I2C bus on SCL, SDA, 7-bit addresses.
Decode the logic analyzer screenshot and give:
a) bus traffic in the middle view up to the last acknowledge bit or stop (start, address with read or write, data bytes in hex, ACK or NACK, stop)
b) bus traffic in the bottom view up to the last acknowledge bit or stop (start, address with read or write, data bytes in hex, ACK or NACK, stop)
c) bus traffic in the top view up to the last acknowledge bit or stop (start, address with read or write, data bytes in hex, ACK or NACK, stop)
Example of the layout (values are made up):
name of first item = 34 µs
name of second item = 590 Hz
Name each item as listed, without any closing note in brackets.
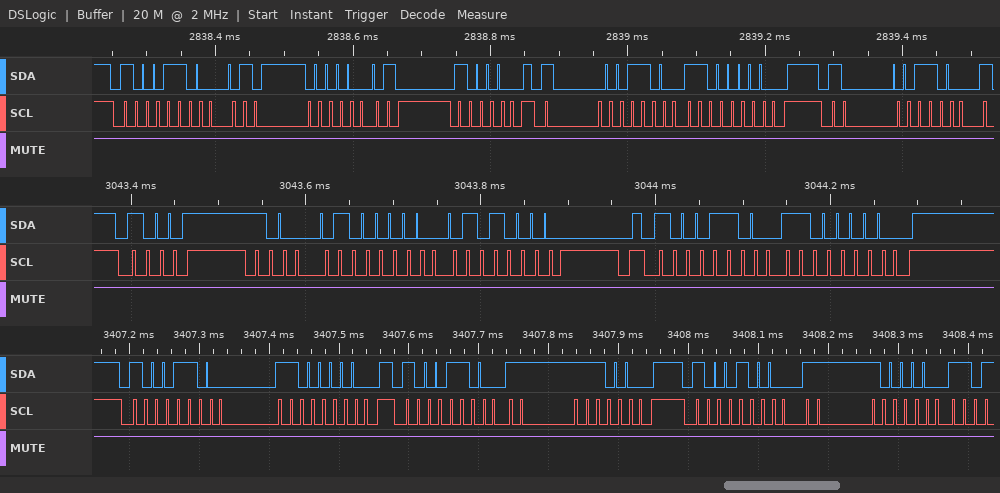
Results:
bus traffic in the middle view up to the last acknowledge bit or stop = start, address 46 write ACK, 40 ACK, 50 ACK, stop, start, address 46 write ACK, C0 ACK, stop
bus traffic in the bottom view up to the last acknowledge bit or stop = start, address 46 write ACK, C0 ACK, stop, start, address 46 write ACK, F8 ACK, stop, start, address 44 write ACK, E0 ACK
bus traffic in the top view up to the last acknowledge bit or stop = start, address 46 write ACK, 40 ACK, 50 ACK, stop, start, address 46 write ACK, C0 ACK, stop, start, address 46 write ACK
